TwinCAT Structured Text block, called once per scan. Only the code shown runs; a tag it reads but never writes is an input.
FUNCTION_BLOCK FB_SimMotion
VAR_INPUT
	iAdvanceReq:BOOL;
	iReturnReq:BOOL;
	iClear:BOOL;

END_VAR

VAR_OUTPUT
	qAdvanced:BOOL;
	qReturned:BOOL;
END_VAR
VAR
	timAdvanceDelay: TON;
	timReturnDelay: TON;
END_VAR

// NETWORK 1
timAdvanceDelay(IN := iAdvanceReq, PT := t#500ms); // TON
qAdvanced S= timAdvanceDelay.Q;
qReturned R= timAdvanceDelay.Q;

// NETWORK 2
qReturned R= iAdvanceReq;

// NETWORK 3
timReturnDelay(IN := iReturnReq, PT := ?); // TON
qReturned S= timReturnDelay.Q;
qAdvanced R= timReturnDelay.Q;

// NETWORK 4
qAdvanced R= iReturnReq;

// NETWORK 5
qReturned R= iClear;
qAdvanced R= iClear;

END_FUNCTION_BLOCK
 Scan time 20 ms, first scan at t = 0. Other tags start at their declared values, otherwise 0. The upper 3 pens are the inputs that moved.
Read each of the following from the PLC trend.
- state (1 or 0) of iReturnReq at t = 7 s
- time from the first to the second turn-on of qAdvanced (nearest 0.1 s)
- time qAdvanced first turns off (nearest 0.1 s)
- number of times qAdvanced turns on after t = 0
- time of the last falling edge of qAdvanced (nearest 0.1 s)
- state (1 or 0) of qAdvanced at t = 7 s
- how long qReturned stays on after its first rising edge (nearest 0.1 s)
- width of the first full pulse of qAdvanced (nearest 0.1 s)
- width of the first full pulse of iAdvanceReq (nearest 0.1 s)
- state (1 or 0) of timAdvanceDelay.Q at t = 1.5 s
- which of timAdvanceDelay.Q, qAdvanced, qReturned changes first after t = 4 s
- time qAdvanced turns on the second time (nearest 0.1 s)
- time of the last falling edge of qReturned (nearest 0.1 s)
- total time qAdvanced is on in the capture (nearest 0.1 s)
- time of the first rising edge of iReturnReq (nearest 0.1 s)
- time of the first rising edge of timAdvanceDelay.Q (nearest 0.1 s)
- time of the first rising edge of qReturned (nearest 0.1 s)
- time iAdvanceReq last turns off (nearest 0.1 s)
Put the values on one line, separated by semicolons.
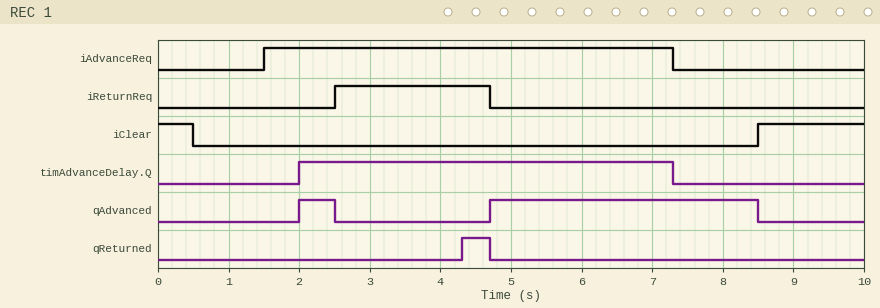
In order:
0; 2.7 s; 2.5 s; 2; 8.5 s; 1; 0.4 s; 0.5 s; 5.8 s; 0; qReturned; 4.7 s; 4.7 s; 4.3 s; 2.5 s; 2.0 s; 4.3 s; 7.3 s
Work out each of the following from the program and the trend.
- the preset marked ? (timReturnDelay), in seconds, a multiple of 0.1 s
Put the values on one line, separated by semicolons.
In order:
1.8 s
